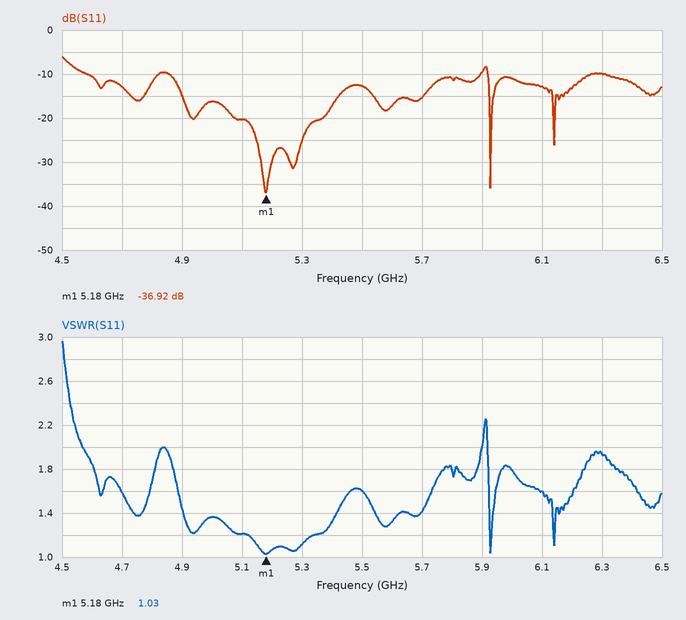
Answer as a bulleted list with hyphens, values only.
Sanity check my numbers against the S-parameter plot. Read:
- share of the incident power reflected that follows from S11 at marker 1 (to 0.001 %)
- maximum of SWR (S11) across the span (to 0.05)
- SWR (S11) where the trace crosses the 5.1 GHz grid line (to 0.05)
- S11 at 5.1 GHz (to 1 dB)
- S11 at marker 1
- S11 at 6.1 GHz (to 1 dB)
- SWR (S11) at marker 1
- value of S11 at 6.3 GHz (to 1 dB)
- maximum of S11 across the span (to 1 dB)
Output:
- 0.020 %
- 2.95
- 1.20
- -20 dB
- -36.92 dB
- -13 dB
- 1.03
- -10 dB
- -6 dB
